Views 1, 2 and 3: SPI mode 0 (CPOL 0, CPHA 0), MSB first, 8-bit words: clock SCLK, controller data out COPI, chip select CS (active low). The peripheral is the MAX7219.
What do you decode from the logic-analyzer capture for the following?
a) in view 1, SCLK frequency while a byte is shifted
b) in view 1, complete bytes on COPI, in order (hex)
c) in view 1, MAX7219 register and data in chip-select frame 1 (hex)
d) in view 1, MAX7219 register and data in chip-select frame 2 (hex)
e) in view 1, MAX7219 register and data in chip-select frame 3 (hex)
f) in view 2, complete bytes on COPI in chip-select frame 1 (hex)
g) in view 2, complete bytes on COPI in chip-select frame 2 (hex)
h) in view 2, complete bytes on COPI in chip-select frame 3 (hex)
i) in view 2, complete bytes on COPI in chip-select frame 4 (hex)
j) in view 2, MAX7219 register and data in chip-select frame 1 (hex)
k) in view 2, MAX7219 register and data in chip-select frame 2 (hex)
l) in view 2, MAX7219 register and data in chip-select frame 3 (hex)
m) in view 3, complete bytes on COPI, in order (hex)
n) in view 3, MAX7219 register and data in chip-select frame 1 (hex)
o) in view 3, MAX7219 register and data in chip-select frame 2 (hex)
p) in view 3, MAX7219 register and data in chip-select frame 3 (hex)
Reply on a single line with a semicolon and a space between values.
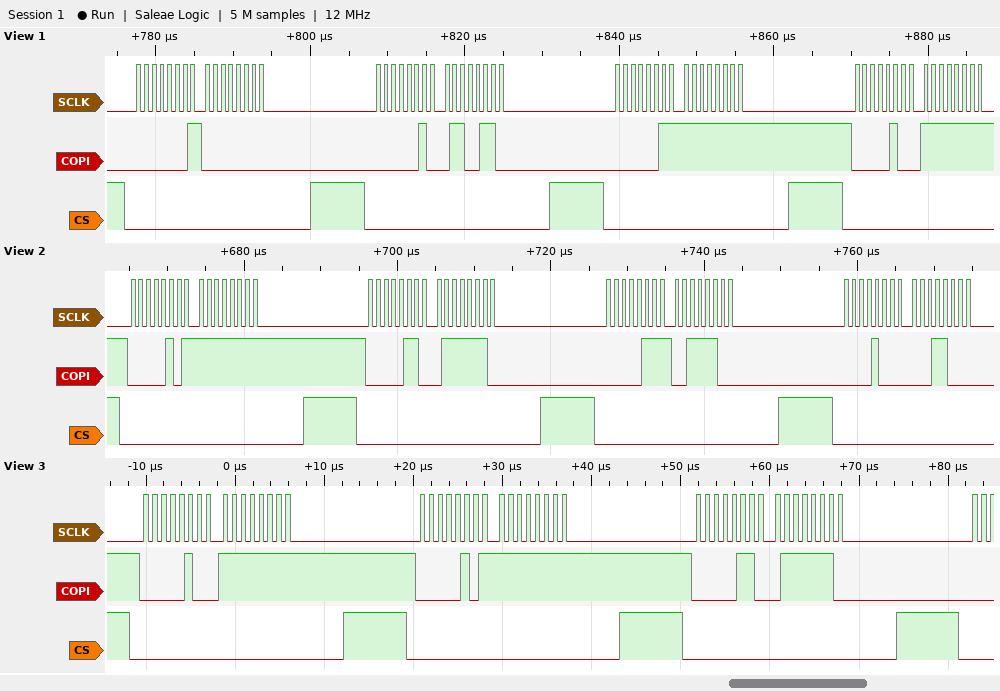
1 MHz; 01 00 02 66 03 FF 04 FF; register 0x1, data 0x00; register 0x2, data 0x66; register 0x3, data 0xFF; 05 FF; 06 7E; 07 3C; 08 18; register 0x5, data 0xFF; register 0x6, data 0x7E; register 0x7, data 0x3C; 04 FF 05 FF 06 7E; register 0x4, data 0xFF; register 0x5, data 0xFF; register 0x6, data 0x7E
